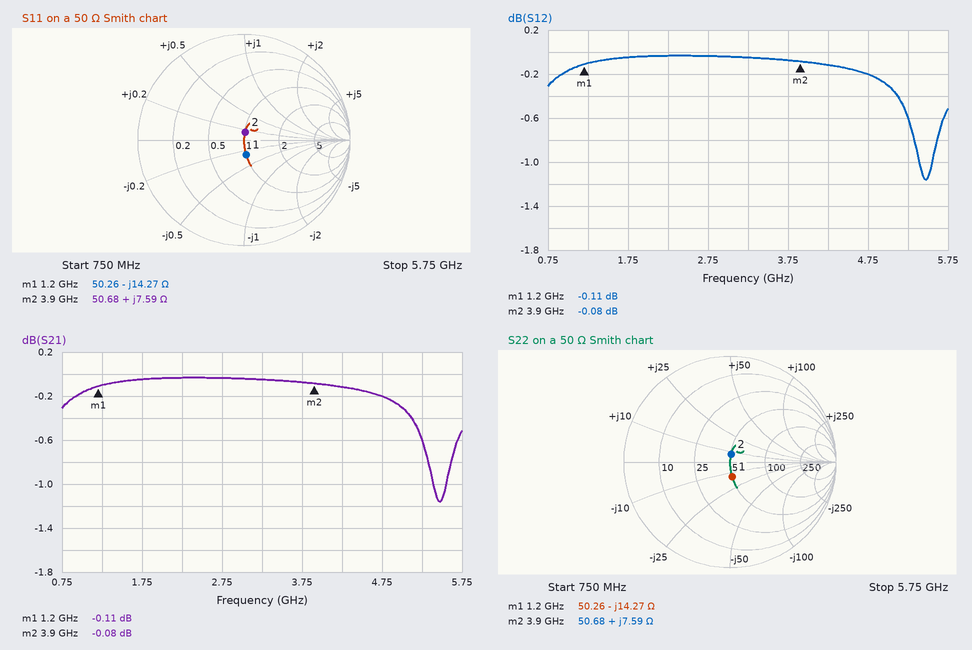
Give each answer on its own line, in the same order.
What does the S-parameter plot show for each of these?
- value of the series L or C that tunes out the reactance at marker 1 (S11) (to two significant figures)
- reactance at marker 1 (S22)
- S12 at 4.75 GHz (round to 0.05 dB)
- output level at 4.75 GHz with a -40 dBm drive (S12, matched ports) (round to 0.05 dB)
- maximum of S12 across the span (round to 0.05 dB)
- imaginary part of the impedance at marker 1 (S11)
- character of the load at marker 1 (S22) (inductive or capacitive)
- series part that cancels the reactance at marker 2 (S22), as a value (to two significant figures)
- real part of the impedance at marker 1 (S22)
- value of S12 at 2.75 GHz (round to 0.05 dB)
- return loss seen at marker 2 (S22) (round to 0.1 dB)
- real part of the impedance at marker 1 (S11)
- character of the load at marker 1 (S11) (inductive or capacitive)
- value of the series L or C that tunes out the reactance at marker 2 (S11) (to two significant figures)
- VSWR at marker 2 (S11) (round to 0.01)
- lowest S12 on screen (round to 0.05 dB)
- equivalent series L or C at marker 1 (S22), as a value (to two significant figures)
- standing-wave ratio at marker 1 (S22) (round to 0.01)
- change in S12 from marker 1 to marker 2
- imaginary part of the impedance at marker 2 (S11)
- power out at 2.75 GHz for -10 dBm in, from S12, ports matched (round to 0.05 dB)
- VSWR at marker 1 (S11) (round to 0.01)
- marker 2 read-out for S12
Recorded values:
1.9 nH
-14.27 Ω
-0.20 dB
-40.20 dBm
-0.05 dB
-14.27 Ω
capacitive
5.4 pF
50.26 Ω
-0.05 dB
22.4 dB
50.26 Ω
capacitive
5.4 pF
1.16
-1.15 dB
9.3 pF
1.33
0.03 dB
+7.59 Ω
-10.05 dBm
1.33
-0.08 dB
